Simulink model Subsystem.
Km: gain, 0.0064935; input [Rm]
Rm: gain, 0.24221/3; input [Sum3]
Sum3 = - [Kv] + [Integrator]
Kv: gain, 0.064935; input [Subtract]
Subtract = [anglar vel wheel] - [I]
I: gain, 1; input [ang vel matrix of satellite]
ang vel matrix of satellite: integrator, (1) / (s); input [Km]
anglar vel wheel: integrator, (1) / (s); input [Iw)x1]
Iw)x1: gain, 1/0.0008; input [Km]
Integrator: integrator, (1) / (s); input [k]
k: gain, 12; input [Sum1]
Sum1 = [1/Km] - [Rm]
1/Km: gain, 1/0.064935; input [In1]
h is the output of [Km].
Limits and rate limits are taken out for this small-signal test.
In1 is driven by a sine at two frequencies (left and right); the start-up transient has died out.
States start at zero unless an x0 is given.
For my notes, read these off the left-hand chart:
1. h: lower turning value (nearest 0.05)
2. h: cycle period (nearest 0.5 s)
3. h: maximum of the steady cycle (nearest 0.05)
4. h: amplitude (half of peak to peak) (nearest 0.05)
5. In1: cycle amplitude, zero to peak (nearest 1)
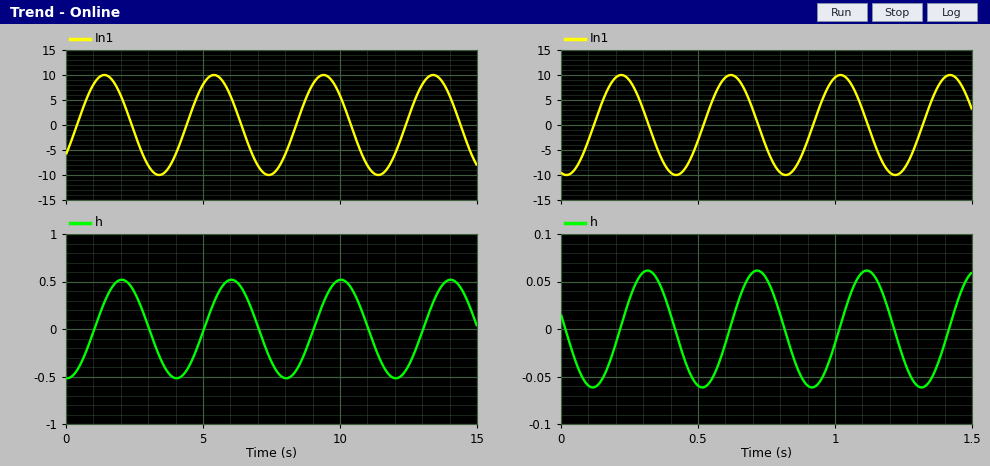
-0.50
4.0 s
0.50
0.50
10
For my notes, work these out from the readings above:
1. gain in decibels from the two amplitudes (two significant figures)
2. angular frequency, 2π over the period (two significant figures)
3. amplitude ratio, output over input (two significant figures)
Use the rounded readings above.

-26 dB
1.6 rad/s
0.050
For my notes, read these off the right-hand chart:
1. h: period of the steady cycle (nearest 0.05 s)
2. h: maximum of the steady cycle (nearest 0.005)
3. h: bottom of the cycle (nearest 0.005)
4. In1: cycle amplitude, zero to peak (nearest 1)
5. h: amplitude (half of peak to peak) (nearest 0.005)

0.40 s
0.060
-0.060
10
0.060
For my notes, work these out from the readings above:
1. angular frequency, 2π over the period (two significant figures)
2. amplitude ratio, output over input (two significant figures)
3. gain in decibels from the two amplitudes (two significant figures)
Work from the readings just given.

16 rad/s
0.0060
-44 dB
